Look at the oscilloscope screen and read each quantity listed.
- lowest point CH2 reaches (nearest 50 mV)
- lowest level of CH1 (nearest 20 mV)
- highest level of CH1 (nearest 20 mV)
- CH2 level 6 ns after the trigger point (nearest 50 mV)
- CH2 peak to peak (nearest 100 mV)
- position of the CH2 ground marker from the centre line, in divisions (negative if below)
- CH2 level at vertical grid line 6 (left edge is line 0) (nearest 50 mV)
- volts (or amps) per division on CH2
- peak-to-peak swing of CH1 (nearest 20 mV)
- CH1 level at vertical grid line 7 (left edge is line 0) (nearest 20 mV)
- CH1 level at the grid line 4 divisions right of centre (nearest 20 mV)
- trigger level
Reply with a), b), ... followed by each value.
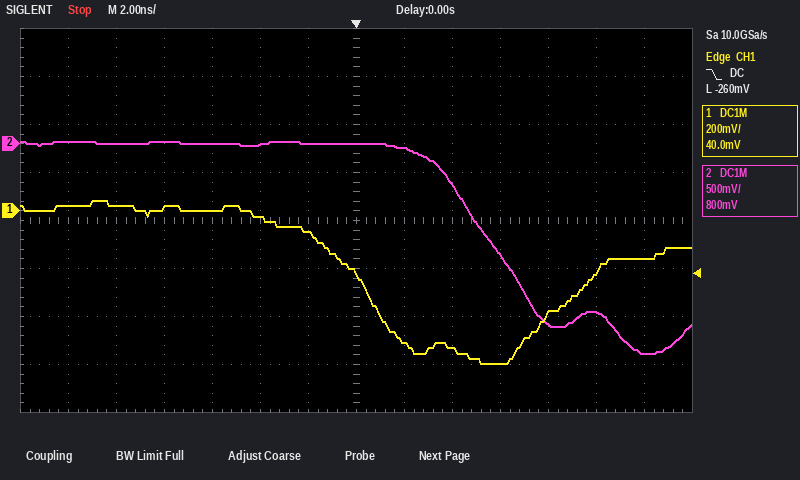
a) -2.20 V
b) -640 mV
c) 40 mV
d) -1.15 V
e) 2.20 V
f) +1.6 div
g) 0 mV
h) 500 mV
i) 680 mV
j) -260 mV
k) -420 mV
l) -260 mV
